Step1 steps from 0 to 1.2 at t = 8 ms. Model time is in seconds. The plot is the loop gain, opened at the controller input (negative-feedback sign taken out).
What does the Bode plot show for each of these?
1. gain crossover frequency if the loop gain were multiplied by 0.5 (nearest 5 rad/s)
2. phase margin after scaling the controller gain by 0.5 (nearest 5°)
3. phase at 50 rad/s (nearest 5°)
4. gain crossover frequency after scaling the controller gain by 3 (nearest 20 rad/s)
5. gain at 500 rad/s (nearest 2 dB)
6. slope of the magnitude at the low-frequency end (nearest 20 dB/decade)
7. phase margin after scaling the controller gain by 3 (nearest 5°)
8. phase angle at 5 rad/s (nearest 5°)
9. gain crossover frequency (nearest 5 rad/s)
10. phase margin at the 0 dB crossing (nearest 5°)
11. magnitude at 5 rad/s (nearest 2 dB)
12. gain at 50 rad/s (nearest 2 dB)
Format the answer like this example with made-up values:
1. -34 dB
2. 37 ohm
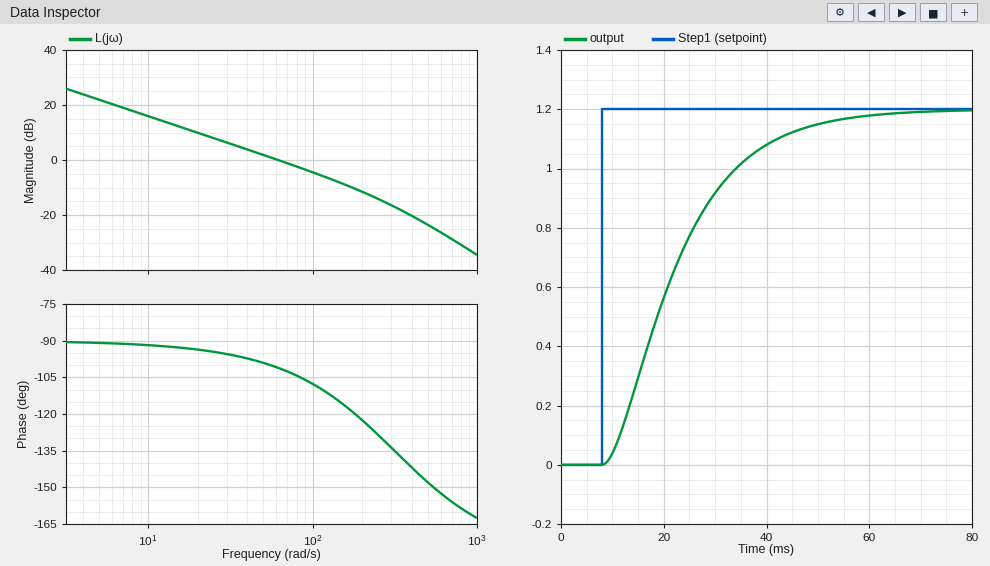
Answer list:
1. 30 rad/s
2. 85°
3. -100°
4. 160 rad/s
5. -24 dB
6. -20 dB/decade
7. 60°
8. -90°
9. 60 rad/s
10. 80°
11. 22 dB
12. 2 dB
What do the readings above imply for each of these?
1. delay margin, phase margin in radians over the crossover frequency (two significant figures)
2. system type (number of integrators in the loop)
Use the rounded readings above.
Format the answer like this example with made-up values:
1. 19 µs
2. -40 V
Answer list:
1. 0.023 s
2. 1
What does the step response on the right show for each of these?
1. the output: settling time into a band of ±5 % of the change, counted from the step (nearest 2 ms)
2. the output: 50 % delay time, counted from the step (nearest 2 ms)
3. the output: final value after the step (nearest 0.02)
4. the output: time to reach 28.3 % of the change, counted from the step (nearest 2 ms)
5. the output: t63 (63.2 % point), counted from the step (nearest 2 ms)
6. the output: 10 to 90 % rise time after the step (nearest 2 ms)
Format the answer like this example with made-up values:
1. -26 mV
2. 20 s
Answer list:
1. 40 ms
2. 12 ms
3. 1.20
4. 8 ms
5. 16 ms
6. 28 ms
